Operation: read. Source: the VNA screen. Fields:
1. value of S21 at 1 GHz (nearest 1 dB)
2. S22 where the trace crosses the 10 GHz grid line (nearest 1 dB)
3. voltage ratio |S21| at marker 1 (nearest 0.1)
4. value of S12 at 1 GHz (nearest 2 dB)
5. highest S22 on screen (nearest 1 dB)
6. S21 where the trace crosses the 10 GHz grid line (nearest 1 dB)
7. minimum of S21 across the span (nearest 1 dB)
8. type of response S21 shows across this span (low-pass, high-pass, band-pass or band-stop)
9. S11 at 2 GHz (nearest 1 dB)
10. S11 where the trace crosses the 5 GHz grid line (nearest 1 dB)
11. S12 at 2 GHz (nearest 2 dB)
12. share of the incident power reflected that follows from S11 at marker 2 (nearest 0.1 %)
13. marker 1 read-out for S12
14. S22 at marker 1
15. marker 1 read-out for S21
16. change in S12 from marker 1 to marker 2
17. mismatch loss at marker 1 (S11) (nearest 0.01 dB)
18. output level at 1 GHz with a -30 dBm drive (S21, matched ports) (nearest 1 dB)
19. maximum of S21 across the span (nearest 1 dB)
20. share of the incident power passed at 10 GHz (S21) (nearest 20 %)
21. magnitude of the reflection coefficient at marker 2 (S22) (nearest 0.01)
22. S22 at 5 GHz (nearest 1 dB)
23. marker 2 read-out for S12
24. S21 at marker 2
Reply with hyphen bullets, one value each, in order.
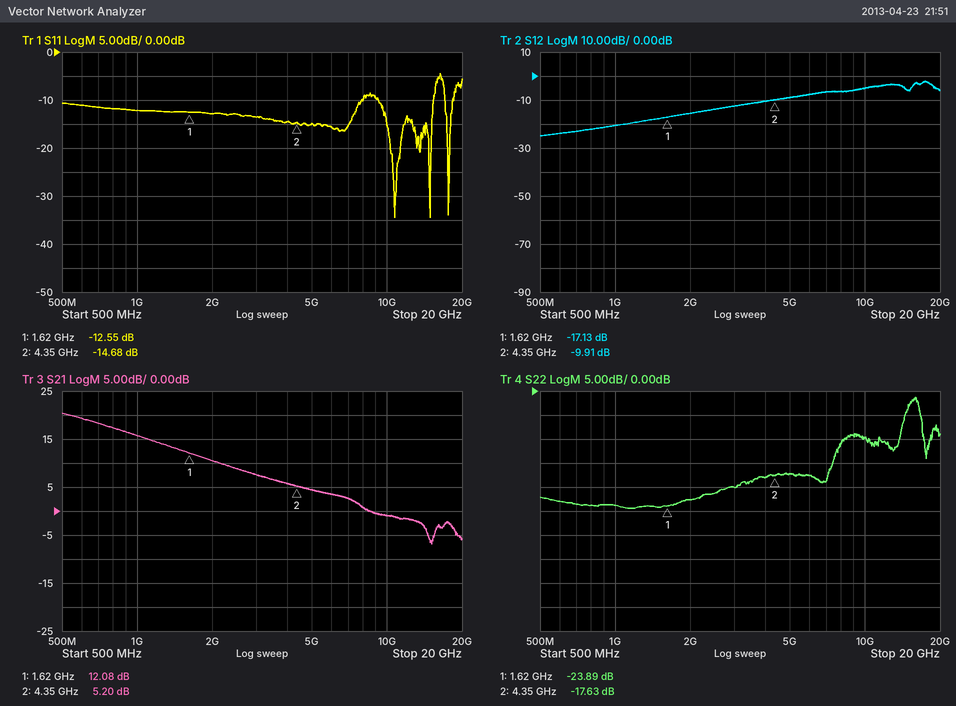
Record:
- 16 dB
- -10 dB
- 4.0
- -20 dB
- -1 dB
- -1 dB
- -7 dB
- low-pass
- -13 dB
- -15 dB
- -16 dB
- 3.4 %
- -17.13 dB
- -23.89 dB
- 12.08 dB
- 7.22 dB
- 0.25 dB
- -14 dBm
- 20 dB
- 80 %
- 0.13
- -17 dB
- -9.91 dB
- 5.20 dB
